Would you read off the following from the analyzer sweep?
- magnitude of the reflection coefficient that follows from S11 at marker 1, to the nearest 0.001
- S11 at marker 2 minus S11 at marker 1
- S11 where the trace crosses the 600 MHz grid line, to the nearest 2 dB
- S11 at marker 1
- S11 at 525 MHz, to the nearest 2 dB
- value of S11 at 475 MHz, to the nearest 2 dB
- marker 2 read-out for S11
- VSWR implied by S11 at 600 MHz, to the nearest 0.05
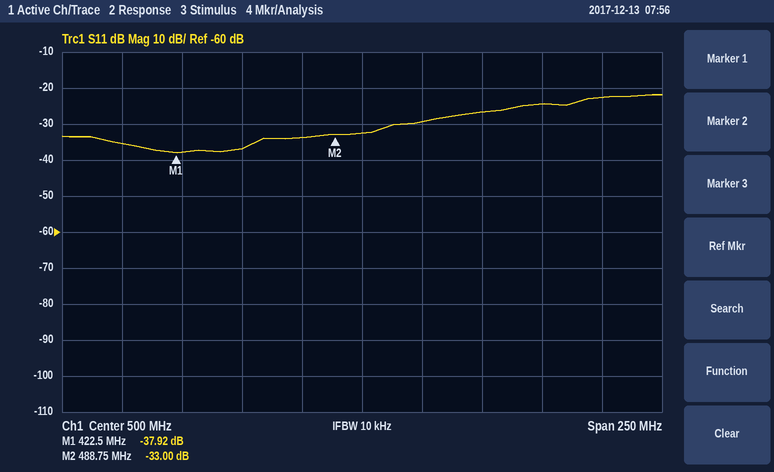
0.013
4.92 dB
-22 dB
-37.92 dB
-30 dB
-34 dB
-33.00 dB
1.15
